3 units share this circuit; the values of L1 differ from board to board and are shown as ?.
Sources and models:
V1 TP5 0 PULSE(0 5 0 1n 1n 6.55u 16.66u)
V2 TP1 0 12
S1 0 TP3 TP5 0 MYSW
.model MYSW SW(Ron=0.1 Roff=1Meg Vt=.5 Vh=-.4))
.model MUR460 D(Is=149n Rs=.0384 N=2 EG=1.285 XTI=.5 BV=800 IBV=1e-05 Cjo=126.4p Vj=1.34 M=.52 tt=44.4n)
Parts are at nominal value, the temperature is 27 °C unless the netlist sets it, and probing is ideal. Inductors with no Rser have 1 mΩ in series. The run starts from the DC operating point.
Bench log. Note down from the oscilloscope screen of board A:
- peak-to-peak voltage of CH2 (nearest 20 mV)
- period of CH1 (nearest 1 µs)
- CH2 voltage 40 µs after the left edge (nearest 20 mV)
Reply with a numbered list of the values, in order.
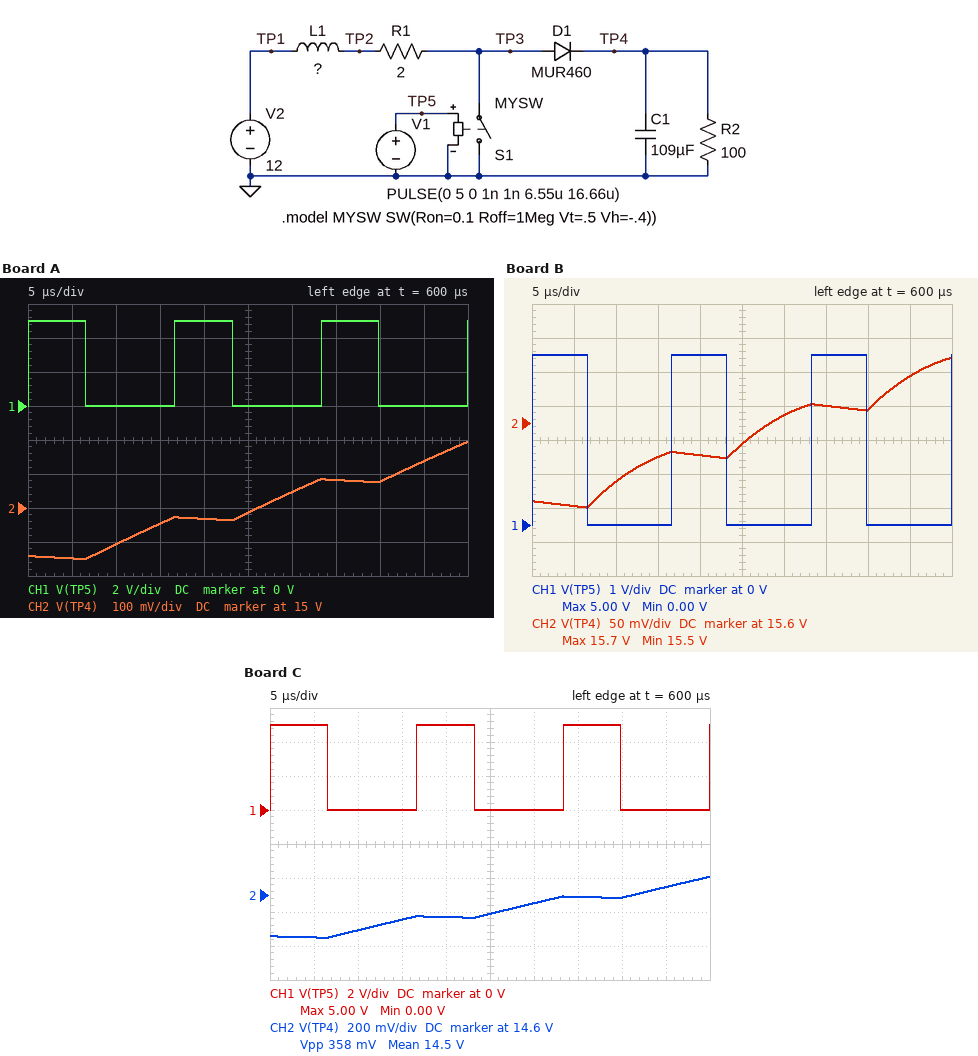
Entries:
1. 340 mV
2. 17 µs
3. 15.08 V
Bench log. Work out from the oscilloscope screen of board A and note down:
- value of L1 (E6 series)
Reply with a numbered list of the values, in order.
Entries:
1. 470 µH
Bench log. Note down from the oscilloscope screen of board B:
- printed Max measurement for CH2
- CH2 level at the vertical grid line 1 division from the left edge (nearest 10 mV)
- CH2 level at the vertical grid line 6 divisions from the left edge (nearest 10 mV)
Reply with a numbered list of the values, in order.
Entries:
1. 15.7 V
2. 15.48 V
3. 15.61 V
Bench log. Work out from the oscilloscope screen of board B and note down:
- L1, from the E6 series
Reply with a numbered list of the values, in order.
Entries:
1. 68 µH
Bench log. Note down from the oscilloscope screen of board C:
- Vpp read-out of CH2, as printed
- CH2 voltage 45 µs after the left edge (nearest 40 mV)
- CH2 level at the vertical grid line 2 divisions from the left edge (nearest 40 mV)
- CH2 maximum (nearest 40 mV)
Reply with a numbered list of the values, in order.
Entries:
1. 358 mV
2. 14.64 V
3. 14.40 V
4. 14.72 V
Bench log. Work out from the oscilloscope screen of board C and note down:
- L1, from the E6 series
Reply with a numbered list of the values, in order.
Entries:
1. 680 µH
